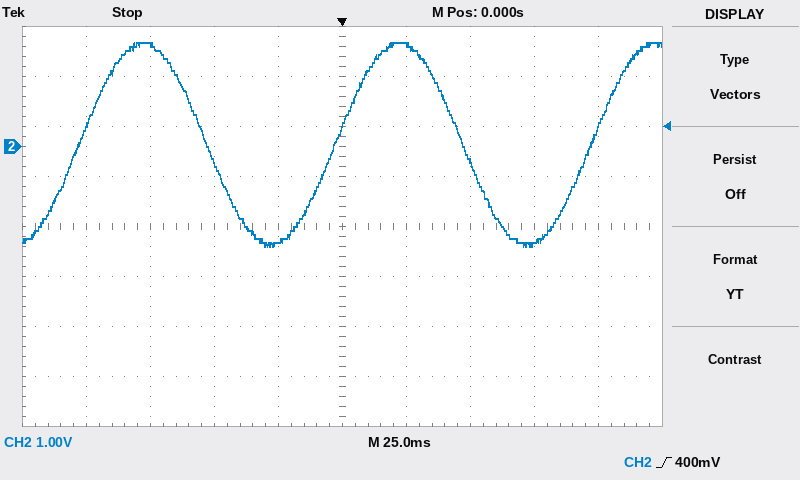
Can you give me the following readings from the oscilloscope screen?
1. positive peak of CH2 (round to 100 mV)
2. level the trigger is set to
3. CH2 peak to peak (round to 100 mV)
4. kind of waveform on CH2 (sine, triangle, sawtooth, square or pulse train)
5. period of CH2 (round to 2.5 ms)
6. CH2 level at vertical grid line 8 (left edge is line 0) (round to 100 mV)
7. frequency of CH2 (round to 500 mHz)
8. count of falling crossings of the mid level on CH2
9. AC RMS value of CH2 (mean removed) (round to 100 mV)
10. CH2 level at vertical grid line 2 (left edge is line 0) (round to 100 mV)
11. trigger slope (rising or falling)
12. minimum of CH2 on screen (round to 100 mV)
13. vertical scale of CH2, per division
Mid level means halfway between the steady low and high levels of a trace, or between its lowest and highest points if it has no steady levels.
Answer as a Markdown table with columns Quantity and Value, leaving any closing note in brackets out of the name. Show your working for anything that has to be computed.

| Quantity | Value |
|---|---|
| positive peak of CH2 | 2.1 V |
| level the trigger is set to | 400 mV |
| CH2 peak to peak | 2.1 V − (-2.0 V) = 4.1 V |
| kind of waveform on CH2 | sine |
| period of CH2 | 100.0 ms |
| CH2 level at vertical grid line 8 (left edge is line 0) | -1.9 V |
| frequency of CH2 | 1 / 100.0 ms ≈ 10.0 Hz |
| count of falling crossings of the mid level on CH2 | 2 |
| AC RMS value of CH2 (mean removed) | 4.1 V / (2√2) ≈ 1.4 V |
| CH2 level at vertical grid line 2 (left edge is line 0) | 2.0 V |
| trigger slope | rising |
| minimum of CH2 on screen | -2.0 V |
| vertical scale of CH2, per division | 1 V |
